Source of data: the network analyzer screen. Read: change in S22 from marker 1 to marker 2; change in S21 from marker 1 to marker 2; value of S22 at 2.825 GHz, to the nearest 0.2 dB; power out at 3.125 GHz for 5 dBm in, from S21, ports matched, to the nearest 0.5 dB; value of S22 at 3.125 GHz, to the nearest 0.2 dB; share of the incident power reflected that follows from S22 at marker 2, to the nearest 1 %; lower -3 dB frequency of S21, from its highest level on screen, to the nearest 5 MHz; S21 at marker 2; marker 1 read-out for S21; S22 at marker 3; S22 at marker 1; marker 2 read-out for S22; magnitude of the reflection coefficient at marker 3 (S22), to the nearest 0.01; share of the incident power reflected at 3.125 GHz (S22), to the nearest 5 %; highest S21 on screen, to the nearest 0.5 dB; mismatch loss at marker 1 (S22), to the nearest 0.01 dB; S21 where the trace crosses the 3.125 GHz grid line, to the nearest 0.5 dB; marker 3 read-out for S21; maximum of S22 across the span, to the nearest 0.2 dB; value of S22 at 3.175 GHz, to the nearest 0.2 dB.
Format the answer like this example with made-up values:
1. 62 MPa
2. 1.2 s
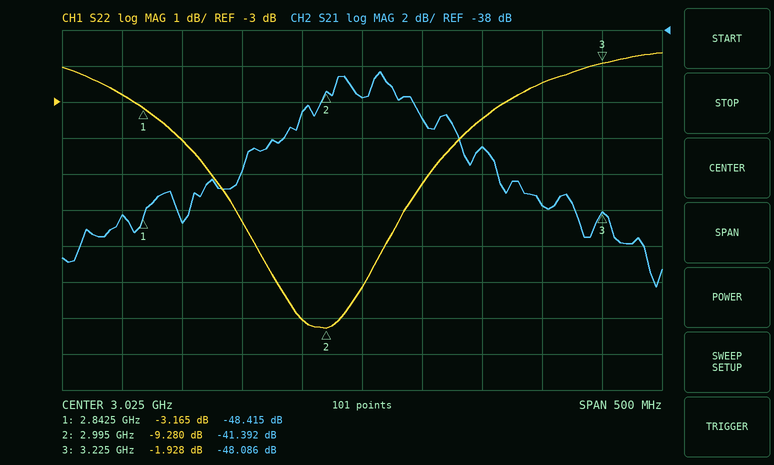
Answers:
1. -6.115 dB
2. 7.023 dB
3. -2.8 dB
4. -39.5 dBm
5. -3.4 dB
6. 12 %
7. 2.970 GHz
8. -41.392 dB
9. -48.415 dB
10. -1.928 dB
11. -3.165 dB
12. -9.280 dB
13. 0.80
14. 45 %
15. -40.5 dB
16. 2.86 dB
17. -44.5 dB
18. -48.086 dB
19. -1.6 dB
20. -2.4 dB
